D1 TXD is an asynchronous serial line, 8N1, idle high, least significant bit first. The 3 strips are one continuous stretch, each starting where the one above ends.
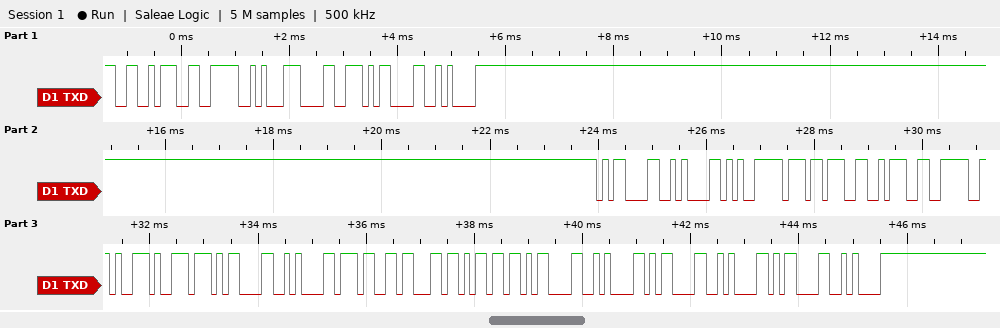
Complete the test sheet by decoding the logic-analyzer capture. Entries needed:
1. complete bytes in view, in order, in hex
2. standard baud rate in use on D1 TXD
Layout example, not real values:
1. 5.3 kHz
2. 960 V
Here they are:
1. A6 E6 8A 98 0D 0A 0D 0A E5 B7 A6 E6 96 B9 0D 0A 37 63 6D 0D 0A 0D 0A 0D 0A
2. 9600 baud
